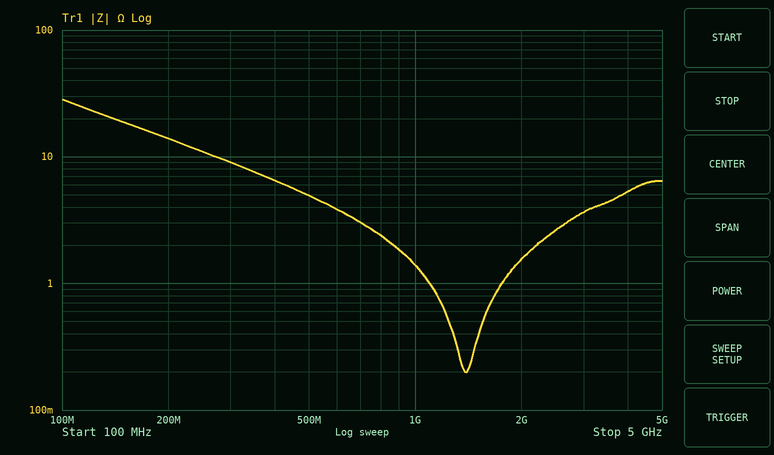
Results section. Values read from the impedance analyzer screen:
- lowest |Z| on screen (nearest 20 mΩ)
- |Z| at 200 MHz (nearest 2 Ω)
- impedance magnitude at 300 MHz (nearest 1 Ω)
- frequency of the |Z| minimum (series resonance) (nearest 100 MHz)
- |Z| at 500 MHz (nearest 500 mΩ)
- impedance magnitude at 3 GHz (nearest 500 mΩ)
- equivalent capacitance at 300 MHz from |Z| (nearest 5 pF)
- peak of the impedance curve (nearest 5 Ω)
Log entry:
200 mΩ
14 Ω
9 Ω
1.4 GHz
5.0 Ω
3.5 Ω
60 pF
30 Ω
